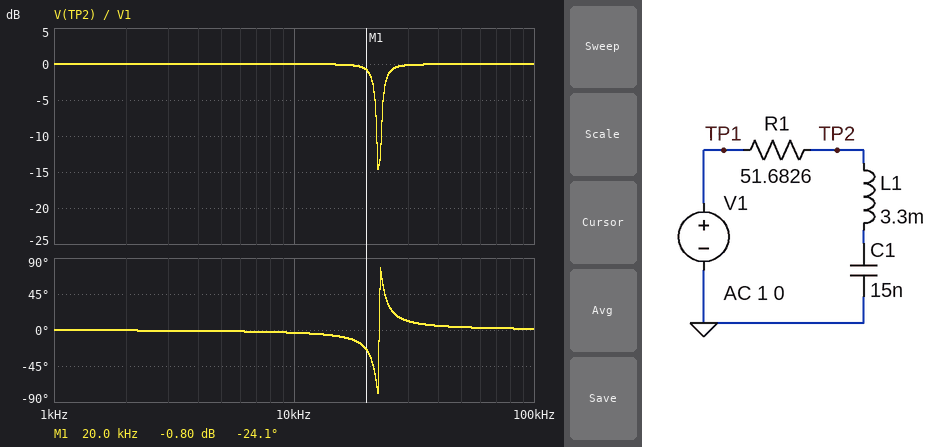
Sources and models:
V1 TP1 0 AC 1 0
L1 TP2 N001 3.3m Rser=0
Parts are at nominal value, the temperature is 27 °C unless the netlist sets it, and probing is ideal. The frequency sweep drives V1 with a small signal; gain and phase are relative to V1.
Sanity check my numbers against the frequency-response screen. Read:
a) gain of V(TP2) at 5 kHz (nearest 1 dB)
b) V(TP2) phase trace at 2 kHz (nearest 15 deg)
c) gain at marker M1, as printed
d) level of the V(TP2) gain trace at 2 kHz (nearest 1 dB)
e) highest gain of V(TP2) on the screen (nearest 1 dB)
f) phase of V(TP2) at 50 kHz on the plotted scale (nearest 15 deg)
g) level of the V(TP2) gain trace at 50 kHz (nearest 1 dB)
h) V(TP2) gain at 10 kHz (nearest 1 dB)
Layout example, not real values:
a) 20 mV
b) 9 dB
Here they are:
a) 0 dB
b) 0 deg
c) -0.80 dB
d) 0 dB
e) 0 dB
f) 0 deg
g) 0 dB
h) 0 dB
